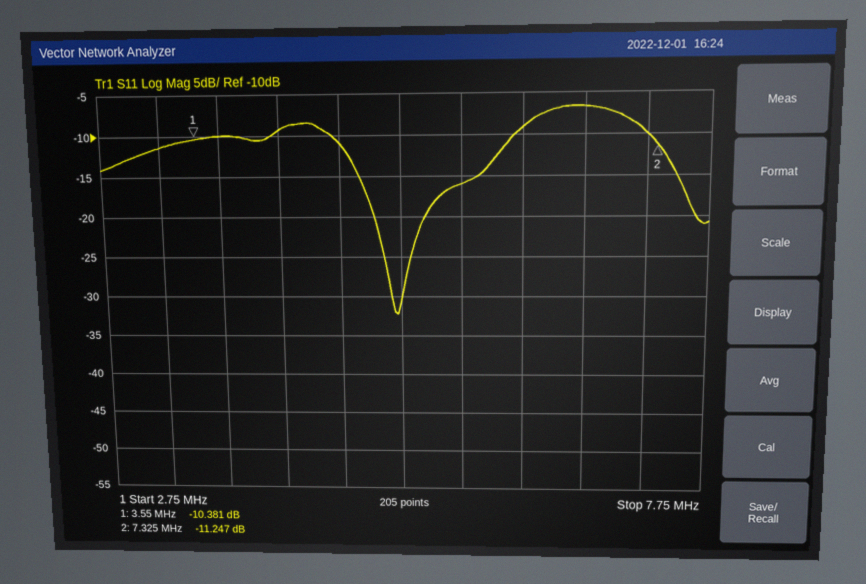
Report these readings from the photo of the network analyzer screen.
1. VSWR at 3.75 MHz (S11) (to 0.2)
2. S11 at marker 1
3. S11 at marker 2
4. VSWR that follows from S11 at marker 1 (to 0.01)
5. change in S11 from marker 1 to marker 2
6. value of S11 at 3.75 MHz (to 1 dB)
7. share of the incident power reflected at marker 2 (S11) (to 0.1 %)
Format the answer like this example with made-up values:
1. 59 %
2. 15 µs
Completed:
1. 2.0
2. -10.381 dB
3. -11.247 dB
4. 1.87
5. -0.866 dB
6. -10 dB
7. 7.5 %
